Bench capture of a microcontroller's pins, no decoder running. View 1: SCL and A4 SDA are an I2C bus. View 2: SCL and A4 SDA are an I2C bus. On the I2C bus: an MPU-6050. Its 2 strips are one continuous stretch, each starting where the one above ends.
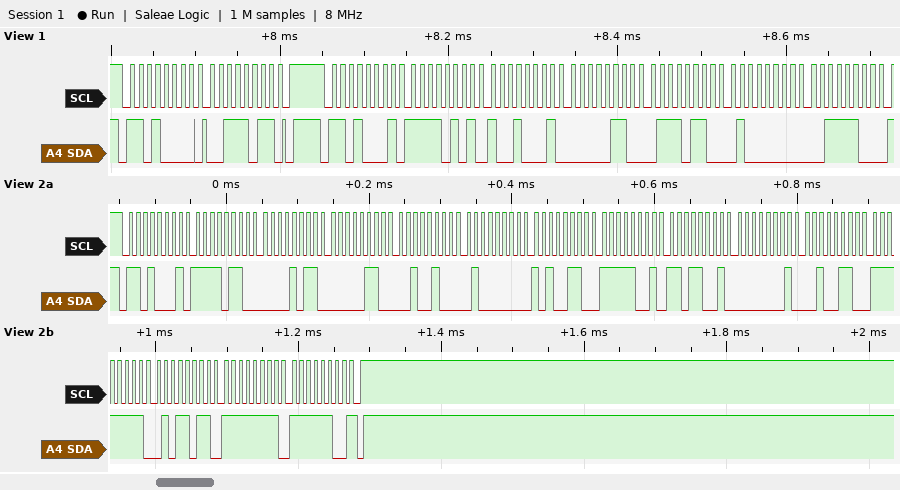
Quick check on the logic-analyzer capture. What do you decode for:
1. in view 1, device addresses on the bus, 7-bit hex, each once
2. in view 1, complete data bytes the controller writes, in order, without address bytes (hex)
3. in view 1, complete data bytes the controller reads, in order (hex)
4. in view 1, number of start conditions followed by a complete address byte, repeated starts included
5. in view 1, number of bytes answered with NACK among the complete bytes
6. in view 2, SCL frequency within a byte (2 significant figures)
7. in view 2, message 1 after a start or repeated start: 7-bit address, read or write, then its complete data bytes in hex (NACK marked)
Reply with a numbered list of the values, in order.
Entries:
1. 0x68
2. 3B
3. F5 91 06 76 40 3C
4. 2
5. 0
6. 100 kHz
7. 0x68 read: F6 0B 06 24 40 A6 F9 D9 01 26 FF 5B FF FC NACK
